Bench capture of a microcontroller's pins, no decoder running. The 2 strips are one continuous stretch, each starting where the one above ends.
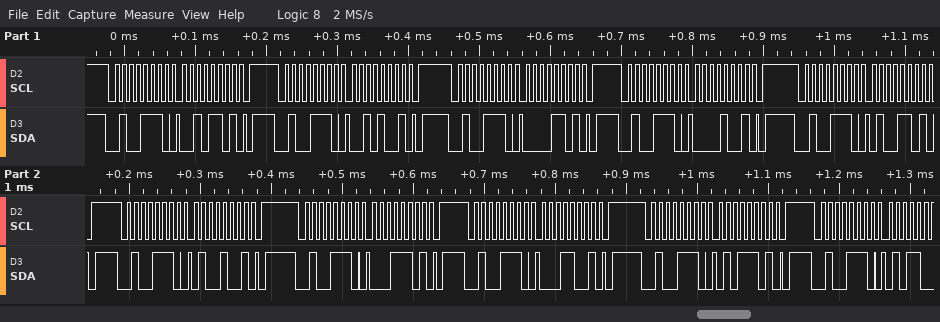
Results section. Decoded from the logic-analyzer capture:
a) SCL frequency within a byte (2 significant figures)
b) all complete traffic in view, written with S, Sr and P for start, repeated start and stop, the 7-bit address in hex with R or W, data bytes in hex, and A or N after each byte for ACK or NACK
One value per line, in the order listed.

100 kHz
S 27W A 2D A P S 27W A 29 A P S 27W A 0D A P S 27W A 09 A P S 27W A 4D A P S 27W A 49 A P S 27W A 1D A P S 27W A 19 A P S 27W A 5D A P S 27W A
